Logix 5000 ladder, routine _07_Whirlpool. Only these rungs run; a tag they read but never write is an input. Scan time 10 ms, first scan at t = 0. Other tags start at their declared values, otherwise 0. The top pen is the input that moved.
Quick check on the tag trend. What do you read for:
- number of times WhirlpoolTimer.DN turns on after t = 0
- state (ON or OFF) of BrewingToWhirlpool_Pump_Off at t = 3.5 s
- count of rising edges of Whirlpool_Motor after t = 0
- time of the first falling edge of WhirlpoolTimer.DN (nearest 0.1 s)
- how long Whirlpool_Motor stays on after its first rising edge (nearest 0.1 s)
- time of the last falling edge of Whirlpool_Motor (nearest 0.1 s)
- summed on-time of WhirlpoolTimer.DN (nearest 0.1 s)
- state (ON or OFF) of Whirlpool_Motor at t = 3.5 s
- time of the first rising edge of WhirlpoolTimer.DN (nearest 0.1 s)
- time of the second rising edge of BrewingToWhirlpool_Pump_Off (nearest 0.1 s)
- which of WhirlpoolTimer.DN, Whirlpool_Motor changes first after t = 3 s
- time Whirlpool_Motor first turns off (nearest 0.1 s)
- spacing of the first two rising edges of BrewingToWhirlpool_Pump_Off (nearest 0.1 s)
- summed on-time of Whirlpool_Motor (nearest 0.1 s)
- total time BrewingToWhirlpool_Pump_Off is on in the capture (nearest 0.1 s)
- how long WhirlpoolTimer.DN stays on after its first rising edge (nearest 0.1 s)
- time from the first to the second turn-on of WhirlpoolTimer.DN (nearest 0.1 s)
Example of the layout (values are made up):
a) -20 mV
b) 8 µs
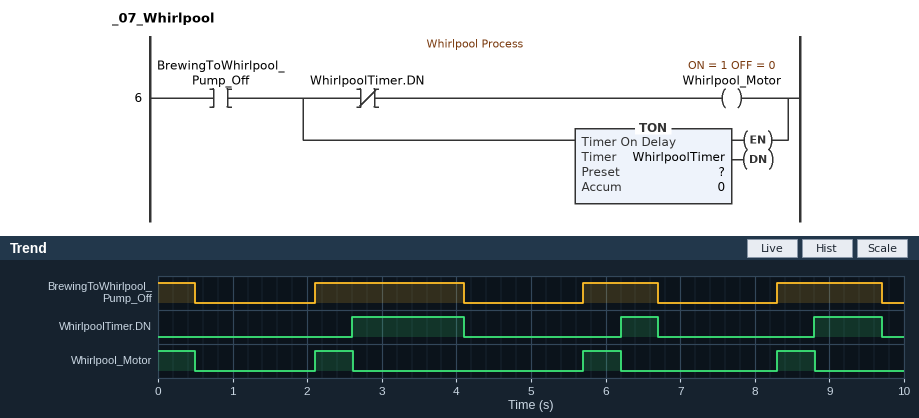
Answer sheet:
a) 3
b) ON
c) 3
d) 4.1 s
e) 0.5 s
f) 8.8 s
g) 2.9 s
h) OFF
i) 2.6 s
j) 5.7 s
k) WhirlpoolTimer.DN
l) 0.5 s
m) 3.6 s
n) 2.0 s
o) 4.9 s
p) 1.5 s
q) 3.6 s
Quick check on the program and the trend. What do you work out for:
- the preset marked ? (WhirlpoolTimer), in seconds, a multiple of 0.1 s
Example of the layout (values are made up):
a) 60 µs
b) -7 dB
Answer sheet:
a) 0.5 s
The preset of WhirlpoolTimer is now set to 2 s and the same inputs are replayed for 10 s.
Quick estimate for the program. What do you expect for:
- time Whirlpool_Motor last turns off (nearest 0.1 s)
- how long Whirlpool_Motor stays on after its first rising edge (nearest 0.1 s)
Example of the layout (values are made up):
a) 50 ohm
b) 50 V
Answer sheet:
a) 9.7 s
b) 2.0 s
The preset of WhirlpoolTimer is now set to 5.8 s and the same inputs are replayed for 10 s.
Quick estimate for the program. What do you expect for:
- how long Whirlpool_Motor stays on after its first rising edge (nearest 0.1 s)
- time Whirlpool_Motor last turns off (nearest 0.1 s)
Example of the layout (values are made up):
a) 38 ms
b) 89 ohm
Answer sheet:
a) 2.0 s
b) 9.7 s
